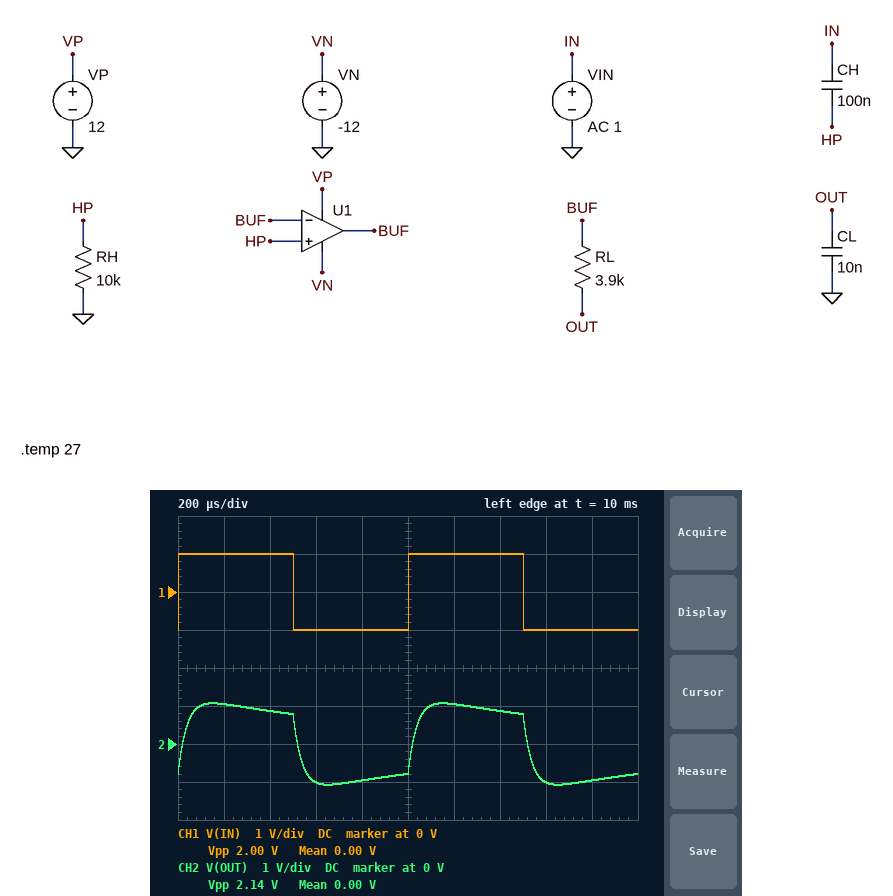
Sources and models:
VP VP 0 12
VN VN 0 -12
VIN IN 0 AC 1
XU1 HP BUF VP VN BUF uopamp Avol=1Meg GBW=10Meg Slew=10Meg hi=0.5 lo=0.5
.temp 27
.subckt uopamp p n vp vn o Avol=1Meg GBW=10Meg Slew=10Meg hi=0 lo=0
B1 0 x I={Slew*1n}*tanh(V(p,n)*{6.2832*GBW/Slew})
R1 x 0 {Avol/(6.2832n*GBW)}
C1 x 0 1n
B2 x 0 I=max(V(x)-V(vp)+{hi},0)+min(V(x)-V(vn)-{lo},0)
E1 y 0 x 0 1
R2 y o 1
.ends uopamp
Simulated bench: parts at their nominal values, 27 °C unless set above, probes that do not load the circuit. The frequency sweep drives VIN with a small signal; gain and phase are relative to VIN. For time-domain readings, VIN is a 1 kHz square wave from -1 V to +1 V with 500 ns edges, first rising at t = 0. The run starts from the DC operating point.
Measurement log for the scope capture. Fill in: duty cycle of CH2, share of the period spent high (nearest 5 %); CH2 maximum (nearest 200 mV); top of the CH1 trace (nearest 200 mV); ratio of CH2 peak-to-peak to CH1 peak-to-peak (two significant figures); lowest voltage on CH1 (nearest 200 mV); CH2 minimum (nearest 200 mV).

50 %
1.0 V
1.0 V
1.1
-1.0 V
-1.0 V
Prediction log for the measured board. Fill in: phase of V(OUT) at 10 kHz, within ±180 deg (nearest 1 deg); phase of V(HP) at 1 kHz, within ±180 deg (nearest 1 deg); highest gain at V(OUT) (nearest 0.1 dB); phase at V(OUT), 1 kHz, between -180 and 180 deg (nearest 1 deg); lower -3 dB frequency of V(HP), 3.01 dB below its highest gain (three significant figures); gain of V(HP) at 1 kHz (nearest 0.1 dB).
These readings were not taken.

-67 deg
9 deg
-0.3 dB
-5 deg
159 Hz
-0.1 dB
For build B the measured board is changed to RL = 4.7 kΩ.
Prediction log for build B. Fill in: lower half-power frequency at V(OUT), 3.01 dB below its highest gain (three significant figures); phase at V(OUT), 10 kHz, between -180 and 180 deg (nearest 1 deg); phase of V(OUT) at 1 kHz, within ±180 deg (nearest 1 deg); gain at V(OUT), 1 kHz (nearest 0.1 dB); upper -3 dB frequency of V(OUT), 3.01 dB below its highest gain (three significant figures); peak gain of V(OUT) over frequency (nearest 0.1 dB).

146 Hz
-70 deg
-7 deg
-0.5 dB
3.69 kHz
-0.4 dB
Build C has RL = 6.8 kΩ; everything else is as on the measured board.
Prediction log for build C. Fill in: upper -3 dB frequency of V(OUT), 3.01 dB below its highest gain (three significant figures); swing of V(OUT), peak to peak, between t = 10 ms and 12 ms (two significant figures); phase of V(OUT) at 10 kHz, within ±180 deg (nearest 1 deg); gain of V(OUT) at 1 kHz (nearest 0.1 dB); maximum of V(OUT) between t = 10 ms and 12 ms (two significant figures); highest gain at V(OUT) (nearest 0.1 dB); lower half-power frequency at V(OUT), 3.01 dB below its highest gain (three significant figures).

2.64 kHz
2.0 V
-76 deg
-0.8 dB
990 mV
-0.6 dB
141 Hz
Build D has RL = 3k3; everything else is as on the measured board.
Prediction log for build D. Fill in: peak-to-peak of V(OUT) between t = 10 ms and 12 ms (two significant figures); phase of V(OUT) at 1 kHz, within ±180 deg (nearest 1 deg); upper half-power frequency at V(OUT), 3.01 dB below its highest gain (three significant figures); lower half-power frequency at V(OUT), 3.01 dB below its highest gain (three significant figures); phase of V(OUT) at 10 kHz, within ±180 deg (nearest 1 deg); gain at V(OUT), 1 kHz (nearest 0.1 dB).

2.2 V
-3 deg
5.13 kHz
150 Hz
-63 deg
-0.3 dB
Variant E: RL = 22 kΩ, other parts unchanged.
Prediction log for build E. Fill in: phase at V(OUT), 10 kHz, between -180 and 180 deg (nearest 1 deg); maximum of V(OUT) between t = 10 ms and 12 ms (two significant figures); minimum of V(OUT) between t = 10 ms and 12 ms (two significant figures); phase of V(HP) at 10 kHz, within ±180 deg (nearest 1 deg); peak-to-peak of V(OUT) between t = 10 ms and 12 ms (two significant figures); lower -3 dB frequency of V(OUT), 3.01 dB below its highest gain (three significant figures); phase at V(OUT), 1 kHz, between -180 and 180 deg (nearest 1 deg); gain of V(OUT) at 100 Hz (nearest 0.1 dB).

-85 deg
730 mV
-730 mV
1 deg
1.5 V
115 Hz
-45 deg
-5.6 dB
